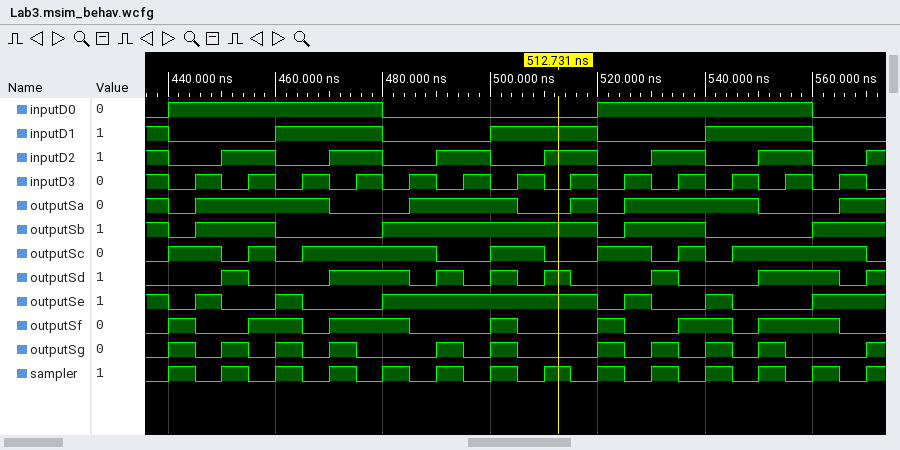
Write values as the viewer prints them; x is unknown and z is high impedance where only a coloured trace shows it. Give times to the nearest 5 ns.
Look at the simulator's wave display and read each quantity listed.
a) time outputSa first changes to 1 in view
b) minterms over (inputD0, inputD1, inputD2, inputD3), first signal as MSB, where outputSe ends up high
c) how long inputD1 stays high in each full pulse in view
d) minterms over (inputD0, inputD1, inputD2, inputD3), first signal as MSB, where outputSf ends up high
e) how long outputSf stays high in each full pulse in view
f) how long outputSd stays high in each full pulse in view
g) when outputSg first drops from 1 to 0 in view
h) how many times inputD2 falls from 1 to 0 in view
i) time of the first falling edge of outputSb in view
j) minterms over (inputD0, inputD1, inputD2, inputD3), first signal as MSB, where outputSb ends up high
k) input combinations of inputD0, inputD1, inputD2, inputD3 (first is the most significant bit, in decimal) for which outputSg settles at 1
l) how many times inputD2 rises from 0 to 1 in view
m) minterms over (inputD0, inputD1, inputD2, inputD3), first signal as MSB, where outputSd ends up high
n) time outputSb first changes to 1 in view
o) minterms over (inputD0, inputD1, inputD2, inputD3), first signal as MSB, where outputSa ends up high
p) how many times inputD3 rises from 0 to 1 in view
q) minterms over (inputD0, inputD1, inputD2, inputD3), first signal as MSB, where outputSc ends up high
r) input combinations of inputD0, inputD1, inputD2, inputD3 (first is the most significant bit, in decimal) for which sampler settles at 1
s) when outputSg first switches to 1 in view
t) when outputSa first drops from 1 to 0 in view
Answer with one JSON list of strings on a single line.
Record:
["445 ns", "0, 1, 2, 3, 4, 5, 6, 7, 9, 12", "20 ns, 20 ns, 20 ns", "0, 4, 8, 11, 12, 14, 15", "5 ns, 10 ns, 15 ns, 5 ns, 5 ns, 10 ns, 15 ns", "5 ns, 15 ns, 5 ns, 5 ns, 5 ns, 5 ns, 15 ns", "445 ns", "7", "440 ns", "0, 1, 2, 3, 4, 5, 6, 7, 9, 10, 11", "2, 4, 8, 10, 12, 14", "7", "0, 2, 4, 6, 10, 14, 15", "445 ns", "1, 2, 3, 4, 7, 9, 10, 11, 12, 13", "13", "0, 1, 4, 5, 8, 9, 11, 13, 14, 15", "0, 2, 4, 6, 8, 10, 12, 14", "440 ns", "440 ns"]
